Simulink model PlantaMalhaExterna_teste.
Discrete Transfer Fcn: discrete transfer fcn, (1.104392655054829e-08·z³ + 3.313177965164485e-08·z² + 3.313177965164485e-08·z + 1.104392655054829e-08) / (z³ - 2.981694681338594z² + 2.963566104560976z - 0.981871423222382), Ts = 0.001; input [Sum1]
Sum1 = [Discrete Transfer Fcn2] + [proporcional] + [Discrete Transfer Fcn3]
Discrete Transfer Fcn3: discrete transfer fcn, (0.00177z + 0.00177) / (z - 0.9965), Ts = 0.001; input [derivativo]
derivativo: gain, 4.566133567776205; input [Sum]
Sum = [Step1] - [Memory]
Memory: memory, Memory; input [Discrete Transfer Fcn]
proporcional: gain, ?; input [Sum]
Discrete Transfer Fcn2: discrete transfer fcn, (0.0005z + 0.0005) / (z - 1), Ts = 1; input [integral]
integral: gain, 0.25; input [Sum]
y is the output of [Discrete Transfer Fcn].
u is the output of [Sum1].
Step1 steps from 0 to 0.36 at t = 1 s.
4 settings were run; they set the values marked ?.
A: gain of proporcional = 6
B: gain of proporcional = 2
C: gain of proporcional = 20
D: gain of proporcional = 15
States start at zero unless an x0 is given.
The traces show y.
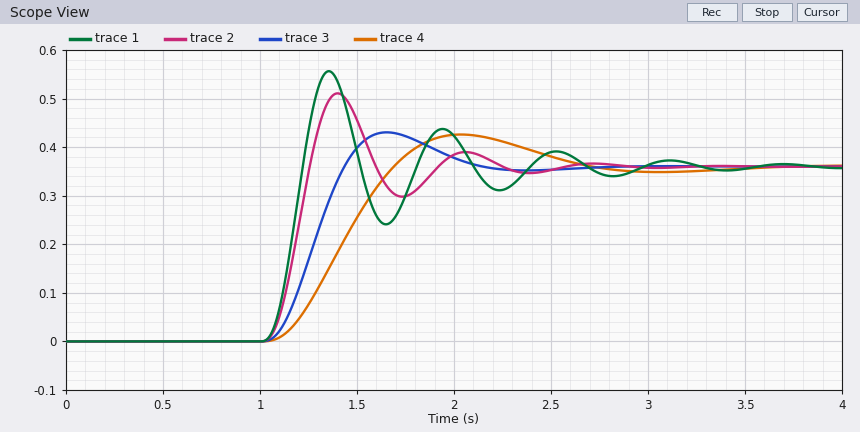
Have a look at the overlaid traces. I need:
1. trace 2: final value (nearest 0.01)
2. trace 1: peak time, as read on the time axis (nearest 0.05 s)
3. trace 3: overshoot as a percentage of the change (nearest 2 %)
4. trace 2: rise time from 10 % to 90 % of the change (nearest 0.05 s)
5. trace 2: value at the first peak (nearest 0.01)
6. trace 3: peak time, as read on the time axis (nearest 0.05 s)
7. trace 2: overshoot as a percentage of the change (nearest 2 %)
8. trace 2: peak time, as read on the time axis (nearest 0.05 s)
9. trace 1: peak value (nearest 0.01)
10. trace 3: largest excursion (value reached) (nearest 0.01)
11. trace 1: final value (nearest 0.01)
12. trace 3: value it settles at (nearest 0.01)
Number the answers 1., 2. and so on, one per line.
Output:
1. 0.36
2. 1.35 s
3. 20 %
4. 0.15 s
5. 0.51
6. 1.65 s
7. 42 %
8. 1.40 s
9. 0.56
10. 0.43
11. 0.36
12. 0.36
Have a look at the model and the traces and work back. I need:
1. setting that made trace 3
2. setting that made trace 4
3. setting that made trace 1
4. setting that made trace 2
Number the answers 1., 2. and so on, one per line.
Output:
1. A
2. B
3. C
4. D
